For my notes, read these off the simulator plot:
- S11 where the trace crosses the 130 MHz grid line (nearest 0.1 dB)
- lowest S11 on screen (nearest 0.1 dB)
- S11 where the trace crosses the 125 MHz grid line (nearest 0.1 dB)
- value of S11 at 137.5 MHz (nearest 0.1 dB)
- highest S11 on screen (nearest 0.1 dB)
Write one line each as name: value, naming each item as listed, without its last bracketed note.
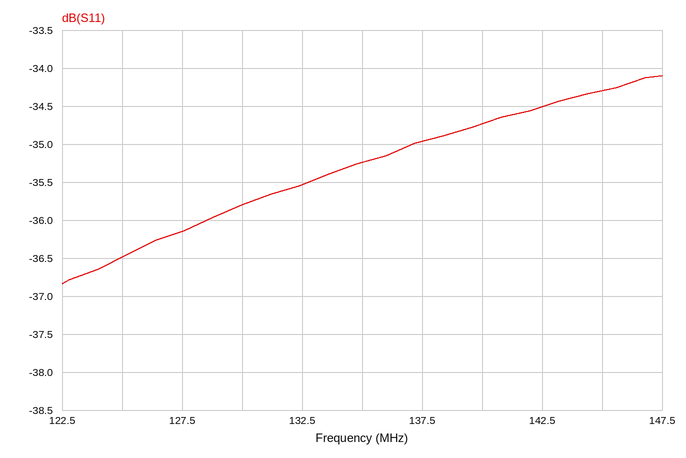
S11 where the trace crosses the 130 MHz grid line: -35.8 dB
lowest S11 on screen: -36.8 dB
S11 where the trace crosses the 125 MHz grid line: -36.5 dB
value of S11 at 137.5 MHz: -35.0 dB
highest S11 on screen: -34.1 dB
